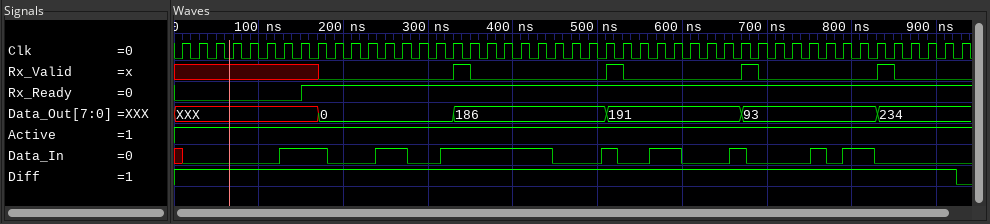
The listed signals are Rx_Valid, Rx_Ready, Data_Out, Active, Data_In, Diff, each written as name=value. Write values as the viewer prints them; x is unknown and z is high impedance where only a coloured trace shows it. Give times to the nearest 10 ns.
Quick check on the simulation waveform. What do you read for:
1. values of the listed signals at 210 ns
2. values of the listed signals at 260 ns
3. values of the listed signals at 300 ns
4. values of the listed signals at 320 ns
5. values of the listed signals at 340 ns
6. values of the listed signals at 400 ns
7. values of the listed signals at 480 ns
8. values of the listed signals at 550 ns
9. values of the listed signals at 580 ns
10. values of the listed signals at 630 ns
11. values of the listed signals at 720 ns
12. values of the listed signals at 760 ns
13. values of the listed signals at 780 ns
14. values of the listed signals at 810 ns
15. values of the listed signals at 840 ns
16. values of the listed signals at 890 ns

Rx_Valid=0, Rx_Ready=1, Data_Out=0, Active=1, Data_In=0, Diff=1
Rx_Valid=0, Rx_Ready=1, Data_Out=0, Active=1, Data_In=1, Diff=1
Rx_Valid=0, Rx_Ready=1, Data_Out=0, Active=1, Data_In=0, Diff=1
Rx_Valid=0, Rx_Ready=1, Data_Out=0, Active=1, Data_In=1, Diff=1
Rx_Valid=1, Rx_Ready=1, Data_Out=186, Active=1, Data_In=1, Diff=1
Rx_Valid=0, Rx_Ready=1, Data_Out=186, Active=1, Data_In=1, Diff=1
Rx_Valid=0, Rx_Ready=1, Data_Out=186, Active=1, Data_In=0, Diff=1
Rx_Valid=0, Rx_Ready=1, Data_Out=191, Active=1, Data_In=0, Diff=1
Rx_Valid=0, Rx_Ready=1, Data_Out=191, Active=1, Data_In=1, Diff=1
Rx_Valid=0, Rx_Ready=1, Data_Out=191, Active=1, Data_In=0, Diff=1
Rx_Valid=0, Rx_Ready=1, Data_Out=93, Active=1, Data_In=0, Diff=1
Rx_Valid=0, Rx_Ready=1, Data_Out=93, Active=1, Data_In=1, Diff=1
Rx_Valid=0, Rx_Ready=1, Data_Out=93, Active=1, Data_In=0, Diff=1
Rx_Valid=0, Rx_Ready=1, Data_Out=93, Active=1, Data_In=1, Diff=1
Rx_Valid=1, Rx_Ready=1, Data_Out=234, Active=1, Data_In=0, Diff=1
Rx_Valid=0, Rx_Ready=1, Data_Out=234, Active=1, Data_In=0, Diff=1
